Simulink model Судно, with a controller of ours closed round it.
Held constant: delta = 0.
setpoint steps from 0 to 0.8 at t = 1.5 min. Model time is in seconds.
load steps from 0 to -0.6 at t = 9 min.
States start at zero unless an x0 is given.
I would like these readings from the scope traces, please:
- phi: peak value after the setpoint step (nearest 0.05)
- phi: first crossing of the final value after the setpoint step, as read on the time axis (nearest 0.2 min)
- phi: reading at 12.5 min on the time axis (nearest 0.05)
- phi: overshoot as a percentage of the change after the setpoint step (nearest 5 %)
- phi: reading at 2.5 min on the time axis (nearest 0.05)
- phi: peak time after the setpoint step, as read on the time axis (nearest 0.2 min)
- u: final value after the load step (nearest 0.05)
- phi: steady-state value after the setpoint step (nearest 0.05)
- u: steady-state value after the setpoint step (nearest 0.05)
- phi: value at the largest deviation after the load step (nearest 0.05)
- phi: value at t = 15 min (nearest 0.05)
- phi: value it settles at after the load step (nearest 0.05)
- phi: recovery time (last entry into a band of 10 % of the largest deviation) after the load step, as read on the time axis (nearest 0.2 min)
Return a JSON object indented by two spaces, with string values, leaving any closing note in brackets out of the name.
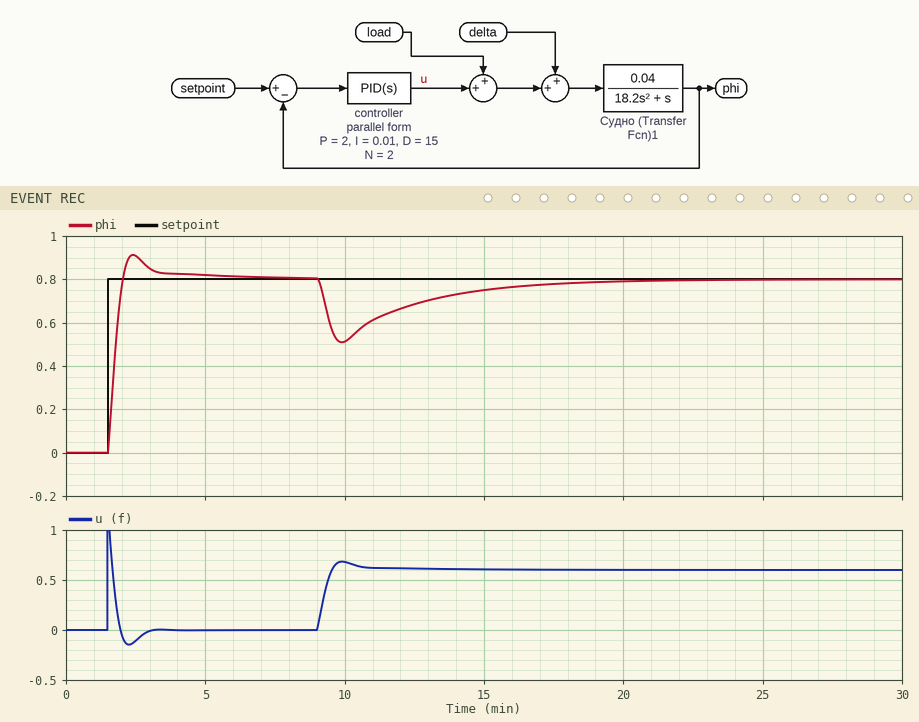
{
  "phi: peak value after the setpoint step": "0.90",
  "phi: first crossing of the final value after the setpoint step, as read on the time axis": "2.0 min",
  "phi: reading at 12.5 min on the time axis": "0.70",
  "phi: overshoot as a percentage of the change after the setpoint step": "15 %",
  "phi: reading at 2.5 min on the time axis": "0.90",
  "phi: peak time after the setpoint step, as read on the time axis": "2.4 min",
  "u: final value after the load step": "0.60",
  "phi: steady-state value after the setpoint step": "0.80",
  "u: steady-state value after the setpoint step": "0.00",
  "phi: value at the largest deviation after the load step": "0.50",
  "phi: value at t = 15 min": "0.75",
  "phi: value it settles at after the load step": "0.80",
  "phi: recovery time (last entry into a band of 10 % of the largest deviation) after the load step, as read on the time axis": "16.6 min"
}
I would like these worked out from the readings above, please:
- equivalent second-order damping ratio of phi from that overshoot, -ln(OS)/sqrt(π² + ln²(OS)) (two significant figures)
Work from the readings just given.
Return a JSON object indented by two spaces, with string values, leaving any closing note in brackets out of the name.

{
  "equivalent second-order damping ratio of phi from that overshoot, -ln(OS)/sqrt(π² + ln²(OS))": "0.52"
}
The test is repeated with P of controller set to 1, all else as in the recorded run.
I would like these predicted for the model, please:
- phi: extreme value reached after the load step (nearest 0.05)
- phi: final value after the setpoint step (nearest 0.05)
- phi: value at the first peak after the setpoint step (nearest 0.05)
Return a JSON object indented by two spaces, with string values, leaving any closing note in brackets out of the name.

{
  "phi: extreme value reached after the load step": "0.35",
  "phi: final value after the setpoint step": "0.80",
  "phi: value at the first peak after the setpoint step": "0.95"
}
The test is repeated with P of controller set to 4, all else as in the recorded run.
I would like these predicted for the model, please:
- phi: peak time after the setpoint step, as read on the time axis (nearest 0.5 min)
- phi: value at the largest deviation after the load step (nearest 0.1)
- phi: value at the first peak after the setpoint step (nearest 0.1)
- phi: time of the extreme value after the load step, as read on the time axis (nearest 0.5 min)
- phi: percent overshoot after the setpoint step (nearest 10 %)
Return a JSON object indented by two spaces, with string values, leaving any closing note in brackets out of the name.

{
  "phi: peak time after the setpoint step, as read on the time axis": "2.0 min",
  "phi: value at the largest deviation after the load step": "0.6",
  "phi: value at the first peak after the setpoint step": "1.0",
  "phi: time of the extreme value after the load step, as read on the time axis": "9.5 min",
  "phi: percent overshoot after the setpoint step": "20 %"
}
